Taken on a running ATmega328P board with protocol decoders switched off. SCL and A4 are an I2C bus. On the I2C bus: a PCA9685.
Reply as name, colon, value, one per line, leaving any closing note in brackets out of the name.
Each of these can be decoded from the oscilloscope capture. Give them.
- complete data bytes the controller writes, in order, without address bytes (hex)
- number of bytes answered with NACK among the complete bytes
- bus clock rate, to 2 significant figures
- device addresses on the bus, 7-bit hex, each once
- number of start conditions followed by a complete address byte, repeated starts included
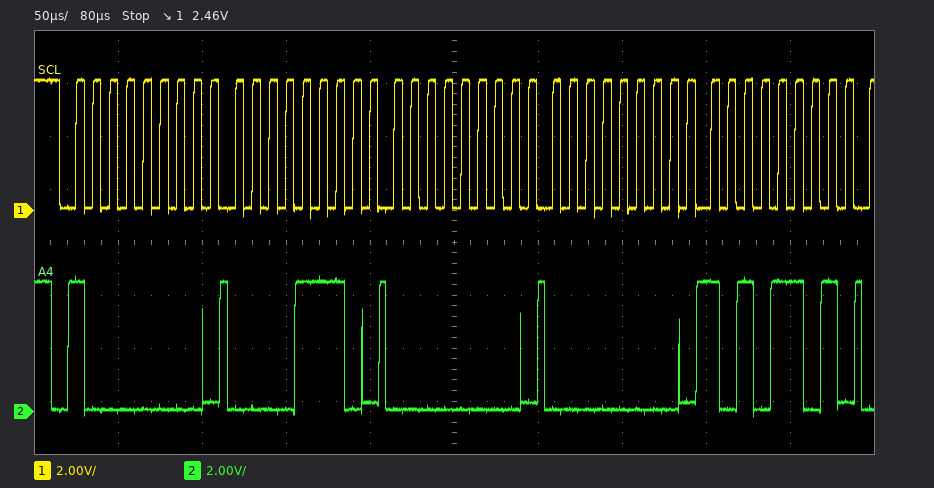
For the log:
complete data bytes the controller writes, in order, without address bytes: 0E 00 00 AD
number of bytes answered with NACK among the complete bytes: 0
bus clock rate, to 2 significant figures: 100 kHz
device addresses on the bus, 7-bit hex, each once: 0x40
number of start conditions followed by a complete address byte, repeated starts included: 1
